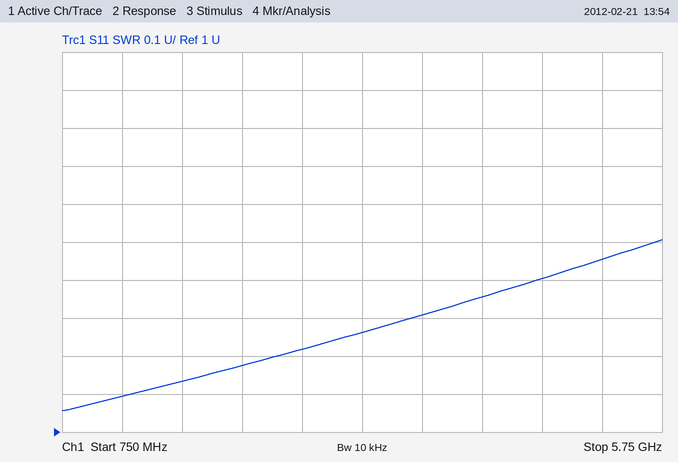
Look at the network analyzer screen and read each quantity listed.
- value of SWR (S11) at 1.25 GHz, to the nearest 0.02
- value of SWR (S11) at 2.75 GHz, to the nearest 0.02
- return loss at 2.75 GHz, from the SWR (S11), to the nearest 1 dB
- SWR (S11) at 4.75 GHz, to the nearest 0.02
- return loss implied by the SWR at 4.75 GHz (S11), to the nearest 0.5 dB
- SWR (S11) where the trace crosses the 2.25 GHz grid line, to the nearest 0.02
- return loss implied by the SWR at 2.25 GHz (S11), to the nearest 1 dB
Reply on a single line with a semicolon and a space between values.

1.10; 1.22; 20 dB; 1.40; 15.5 dB; 1.18; 22 dB
